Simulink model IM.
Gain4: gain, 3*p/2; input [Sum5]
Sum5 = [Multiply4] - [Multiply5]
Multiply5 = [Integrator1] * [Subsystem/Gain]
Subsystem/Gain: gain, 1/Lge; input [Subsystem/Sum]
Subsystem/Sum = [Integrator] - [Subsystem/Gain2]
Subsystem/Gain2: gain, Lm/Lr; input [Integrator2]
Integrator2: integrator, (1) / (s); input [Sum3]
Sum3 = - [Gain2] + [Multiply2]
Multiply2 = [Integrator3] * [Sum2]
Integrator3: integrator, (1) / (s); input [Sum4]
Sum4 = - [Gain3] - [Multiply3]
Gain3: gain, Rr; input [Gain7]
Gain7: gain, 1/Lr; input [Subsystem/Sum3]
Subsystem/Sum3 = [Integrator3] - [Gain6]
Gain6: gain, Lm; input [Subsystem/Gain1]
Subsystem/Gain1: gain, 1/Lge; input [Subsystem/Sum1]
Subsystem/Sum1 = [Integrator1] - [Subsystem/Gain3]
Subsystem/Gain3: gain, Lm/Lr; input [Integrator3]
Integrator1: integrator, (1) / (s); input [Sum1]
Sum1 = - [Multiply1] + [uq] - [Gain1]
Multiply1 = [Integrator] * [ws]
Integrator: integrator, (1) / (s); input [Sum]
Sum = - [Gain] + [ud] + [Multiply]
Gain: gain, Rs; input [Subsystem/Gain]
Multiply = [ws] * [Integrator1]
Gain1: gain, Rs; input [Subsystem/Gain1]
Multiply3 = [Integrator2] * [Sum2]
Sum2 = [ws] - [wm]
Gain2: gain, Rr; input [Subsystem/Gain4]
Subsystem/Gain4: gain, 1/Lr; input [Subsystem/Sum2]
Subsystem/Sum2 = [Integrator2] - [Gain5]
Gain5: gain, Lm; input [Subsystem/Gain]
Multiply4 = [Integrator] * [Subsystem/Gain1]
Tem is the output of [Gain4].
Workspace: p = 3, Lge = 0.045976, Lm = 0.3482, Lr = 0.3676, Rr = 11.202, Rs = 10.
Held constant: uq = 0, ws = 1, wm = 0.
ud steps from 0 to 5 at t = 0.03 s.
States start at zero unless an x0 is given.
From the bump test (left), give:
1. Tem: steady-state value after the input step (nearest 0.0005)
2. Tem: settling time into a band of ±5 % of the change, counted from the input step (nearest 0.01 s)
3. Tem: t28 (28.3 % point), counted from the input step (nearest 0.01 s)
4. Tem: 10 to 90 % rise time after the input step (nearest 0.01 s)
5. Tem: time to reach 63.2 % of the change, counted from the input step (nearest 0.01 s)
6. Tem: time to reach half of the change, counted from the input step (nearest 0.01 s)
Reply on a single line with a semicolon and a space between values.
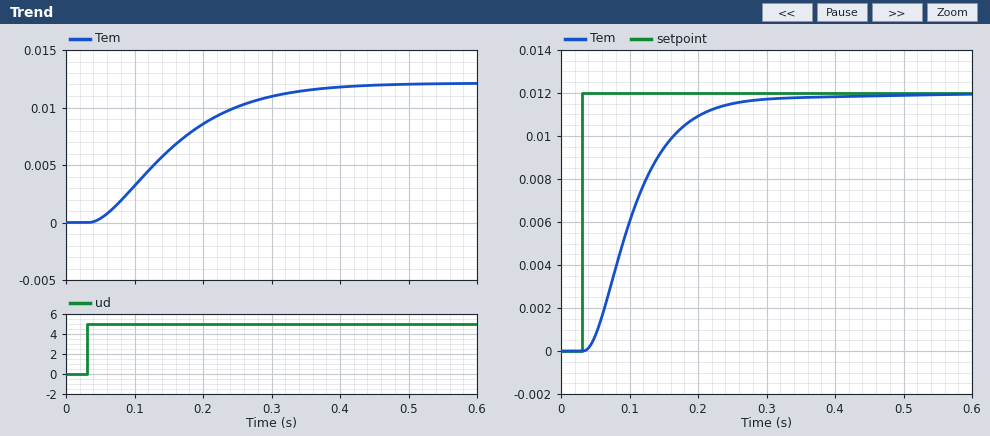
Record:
0.0120; 0.32 s; 0.07 s; 0.23 s; 0.15 s; 0.12 s
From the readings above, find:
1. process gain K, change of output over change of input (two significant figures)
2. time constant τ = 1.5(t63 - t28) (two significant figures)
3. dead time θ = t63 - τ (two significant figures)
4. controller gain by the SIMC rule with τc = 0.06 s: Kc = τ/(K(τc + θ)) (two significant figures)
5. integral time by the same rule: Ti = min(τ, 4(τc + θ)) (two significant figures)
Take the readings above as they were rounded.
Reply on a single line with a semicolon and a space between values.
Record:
0.0024; 0.12 s; 0.030 s; 560; 0.12 s
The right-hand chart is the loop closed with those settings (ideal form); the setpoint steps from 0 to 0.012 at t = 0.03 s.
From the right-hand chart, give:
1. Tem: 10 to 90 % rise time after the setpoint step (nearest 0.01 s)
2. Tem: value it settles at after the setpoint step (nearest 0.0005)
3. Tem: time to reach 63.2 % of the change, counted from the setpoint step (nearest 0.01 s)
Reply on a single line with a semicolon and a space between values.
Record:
0.14 s; 0.0120; 0.09 s
